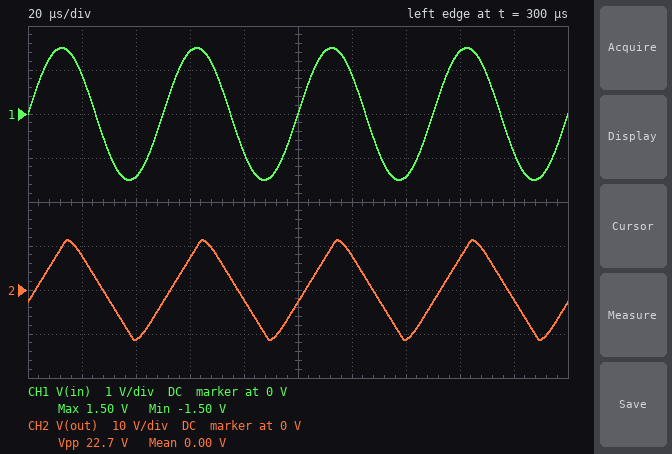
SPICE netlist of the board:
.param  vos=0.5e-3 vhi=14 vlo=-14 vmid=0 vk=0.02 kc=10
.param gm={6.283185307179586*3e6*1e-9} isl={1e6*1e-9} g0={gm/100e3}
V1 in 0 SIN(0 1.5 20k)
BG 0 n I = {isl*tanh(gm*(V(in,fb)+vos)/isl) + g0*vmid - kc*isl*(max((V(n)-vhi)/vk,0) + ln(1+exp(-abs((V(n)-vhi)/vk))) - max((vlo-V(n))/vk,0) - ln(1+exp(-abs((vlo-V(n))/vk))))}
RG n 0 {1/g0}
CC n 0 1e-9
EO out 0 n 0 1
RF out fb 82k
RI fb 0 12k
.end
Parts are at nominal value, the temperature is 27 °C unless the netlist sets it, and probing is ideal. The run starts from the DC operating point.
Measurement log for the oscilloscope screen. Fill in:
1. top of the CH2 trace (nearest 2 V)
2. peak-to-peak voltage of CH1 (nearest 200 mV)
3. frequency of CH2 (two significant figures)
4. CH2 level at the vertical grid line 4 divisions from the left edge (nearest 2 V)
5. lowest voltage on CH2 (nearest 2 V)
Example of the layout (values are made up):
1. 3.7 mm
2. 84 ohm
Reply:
1. 12 V
2. 3.0 V
3. 20 kHz
4. -2 V
5. -12 V
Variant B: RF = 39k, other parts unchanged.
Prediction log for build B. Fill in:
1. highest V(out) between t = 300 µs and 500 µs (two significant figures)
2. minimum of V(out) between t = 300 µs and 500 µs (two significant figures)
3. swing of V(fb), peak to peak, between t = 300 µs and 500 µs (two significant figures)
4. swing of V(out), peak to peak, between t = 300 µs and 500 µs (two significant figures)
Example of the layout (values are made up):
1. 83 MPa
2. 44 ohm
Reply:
1. 6.4 V
2. -6.4 V
3. 3.0 V
4. 13 V
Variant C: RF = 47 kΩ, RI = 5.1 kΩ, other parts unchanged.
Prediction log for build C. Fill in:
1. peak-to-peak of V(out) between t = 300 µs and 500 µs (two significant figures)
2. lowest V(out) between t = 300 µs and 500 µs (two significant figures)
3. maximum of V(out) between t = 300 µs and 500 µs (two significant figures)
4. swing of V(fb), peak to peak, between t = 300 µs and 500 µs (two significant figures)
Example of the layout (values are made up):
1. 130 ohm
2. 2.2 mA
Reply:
1. 24 V
2. -12 V
3. 12 V
4. 2.4 V
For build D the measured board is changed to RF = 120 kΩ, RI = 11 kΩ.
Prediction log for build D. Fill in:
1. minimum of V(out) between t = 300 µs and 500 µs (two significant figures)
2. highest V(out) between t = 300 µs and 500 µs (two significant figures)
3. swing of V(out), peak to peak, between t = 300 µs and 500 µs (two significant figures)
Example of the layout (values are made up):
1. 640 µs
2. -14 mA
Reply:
1. -12 V
2. 12 V
3. 24 V
